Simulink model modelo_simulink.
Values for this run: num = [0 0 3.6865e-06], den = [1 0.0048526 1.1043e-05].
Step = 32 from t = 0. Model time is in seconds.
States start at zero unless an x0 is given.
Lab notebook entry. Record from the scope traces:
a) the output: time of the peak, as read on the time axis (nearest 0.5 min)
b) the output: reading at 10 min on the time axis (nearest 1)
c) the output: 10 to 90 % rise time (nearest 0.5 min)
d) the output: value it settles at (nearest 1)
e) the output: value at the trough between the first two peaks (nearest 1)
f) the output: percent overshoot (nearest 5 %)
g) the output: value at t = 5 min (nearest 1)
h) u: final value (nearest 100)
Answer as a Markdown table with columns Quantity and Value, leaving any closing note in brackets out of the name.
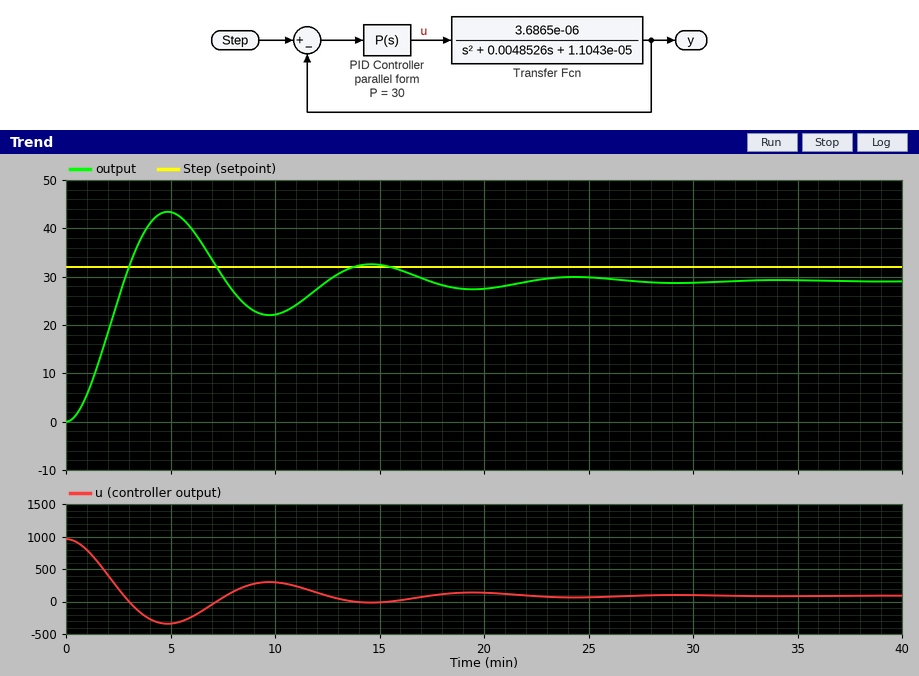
| Quantity | Value |
|---|---|
| the output: time of the peak, as read on the time axis | 5.0 min |
| the output: reading at 10 min on the time axis | 22 |
| the output: 10 to 90 % rise time | 2.0 min |
| the output: value it settles at | 29 |
| the output: value at the trough between the first two peaks | 22 |
| the output: percent overshoot | 50 % |
| the output: value at t = 5 min | 43 |
| u: final value | 100 |
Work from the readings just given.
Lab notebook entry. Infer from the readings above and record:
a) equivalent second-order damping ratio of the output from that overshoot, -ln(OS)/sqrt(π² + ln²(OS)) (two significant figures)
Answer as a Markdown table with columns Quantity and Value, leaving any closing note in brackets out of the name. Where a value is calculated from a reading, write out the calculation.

| Quantity | Value |
|---|---|
| equivalent second-order damping ratio of the output from that overshoot, -ln(OS)/sqrt(π² + ln²(OS)) | ln(0.5) = -0.693; 0.693 / sqrt(9.870 + 0.480) = 0.22 |
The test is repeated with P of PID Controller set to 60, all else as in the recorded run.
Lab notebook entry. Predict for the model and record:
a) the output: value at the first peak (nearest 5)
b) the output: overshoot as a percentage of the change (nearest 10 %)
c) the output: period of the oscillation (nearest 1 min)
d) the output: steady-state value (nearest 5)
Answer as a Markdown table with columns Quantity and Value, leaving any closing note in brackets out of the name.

| Quantity | Value |
|---|---|
| the output: value at the first peak | 50 |
| the output: overshoot as a percentage of the change | 60 % |
| the output: period of the oscillation | 7 min |
| the output: steady-state value | 30 |
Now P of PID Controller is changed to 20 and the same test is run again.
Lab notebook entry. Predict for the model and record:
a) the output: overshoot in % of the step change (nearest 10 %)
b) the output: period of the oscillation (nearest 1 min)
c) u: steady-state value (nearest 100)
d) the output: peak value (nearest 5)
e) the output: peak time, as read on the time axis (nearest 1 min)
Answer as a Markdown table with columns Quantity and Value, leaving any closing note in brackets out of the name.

| Quantity | Value |
|---|---|
| the output: overshoot in % of the step change | 40 % |
| the output: period of the oscillation | 12 min |
| u: steady-state value | 100 |
| the output: peak value | 40 |
| the output: peak time, as read on the time axis | 6 min |
